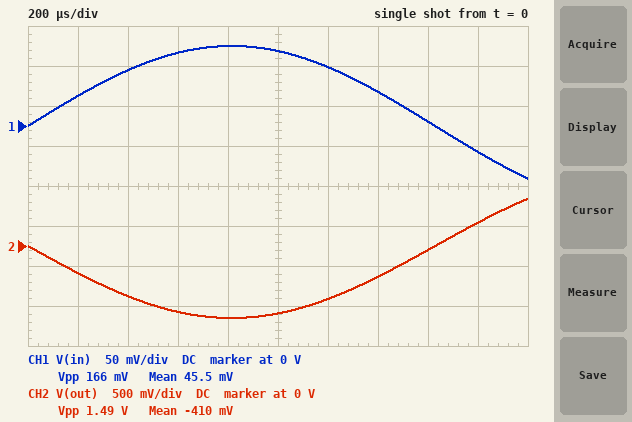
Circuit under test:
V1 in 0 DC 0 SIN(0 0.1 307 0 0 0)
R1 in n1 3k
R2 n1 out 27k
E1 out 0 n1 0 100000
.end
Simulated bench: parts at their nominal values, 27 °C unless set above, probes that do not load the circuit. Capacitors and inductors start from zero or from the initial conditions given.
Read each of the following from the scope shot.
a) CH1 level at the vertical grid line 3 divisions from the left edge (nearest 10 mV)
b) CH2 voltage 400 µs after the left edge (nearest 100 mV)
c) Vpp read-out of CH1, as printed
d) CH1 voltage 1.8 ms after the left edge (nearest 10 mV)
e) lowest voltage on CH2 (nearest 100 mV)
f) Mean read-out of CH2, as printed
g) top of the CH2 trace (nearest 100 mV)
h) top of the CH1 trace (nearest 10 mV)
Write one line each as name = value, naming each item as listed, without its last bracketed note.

CH1 level at the vertical grid line 3 divisions from the left edge = 90 mV
CH2 voltage 400 µs after the left edge = -600 mV
Vpp read-out of CH1, as printed = 166 mV
CH1 voltage 1.8 ms after the left edge = -30 mV
lowest voltage on CH2 = -900 mV
Mean read-out of CH2, as printed = -410 mV
top of the CH2 trace = 600 mV
top of the CH1 trace = 100 mV
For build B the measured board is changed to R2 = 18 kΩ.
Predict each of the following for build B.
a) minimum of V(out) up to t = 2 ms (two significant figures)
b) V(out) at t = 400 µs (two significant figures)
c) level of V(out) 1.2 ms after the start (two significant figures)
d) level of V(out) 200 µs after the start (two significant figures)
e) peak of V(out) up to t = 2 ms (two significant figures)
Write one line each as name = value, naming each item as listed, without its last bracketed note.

minimum of V(out) up to t = 2 ms = -600 mV
V(out) at t = 400 µs = -420 mV
level of V(out) 1.2 ms after the start = -440 mV
level of V(out) 200 µs after the start = -230 mV
peak of V(out) up to t = 2 ms = 390 mV
